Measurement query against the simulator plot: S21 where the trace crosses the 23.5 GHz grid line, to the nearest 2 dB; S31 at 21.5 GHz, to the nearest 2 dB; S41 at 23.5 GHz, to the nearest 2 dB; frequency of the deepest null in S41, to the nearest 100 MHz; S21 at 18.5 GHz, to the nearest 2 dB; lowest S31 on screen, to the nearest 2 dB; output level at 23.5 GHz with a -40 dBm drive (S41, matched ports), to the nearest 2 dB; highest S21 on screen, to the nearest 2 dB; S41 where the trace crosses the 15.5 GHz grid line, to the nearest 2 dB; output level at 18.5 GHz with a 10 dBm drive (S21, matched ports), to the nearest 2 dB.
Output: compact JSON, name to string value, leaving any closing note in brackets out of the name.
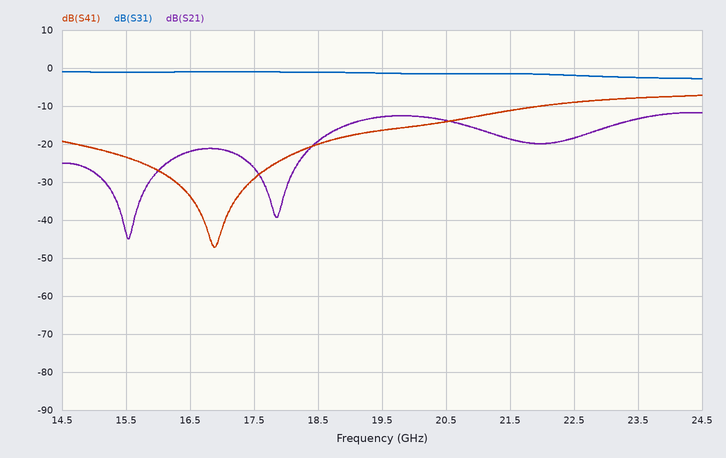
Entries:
{"S21 where the trace crosses the 23.5 GHz grid line, to the nearest 2 dB": "-14 dB", "S31 at 21.5 GHz, to the nearest 2 dB": "-2 dB", "S41 at 23.5 GHz, to the nearest 2 dB": "-8 dB", "frequency of the deepest null in S41, to the nearest 100 MHz": "16.9 GHz", "S21 at 18.5 GHz, to the nearest 2 dB": "-20 dB", "lowest S31 on screen, to the nearest 2 dB": "-2 dB", "output level at 23.5 GHz with a -40 dBm drive (S41, matched ports), to the nearest 2 dB": "-48 dBm", "highest S21 on screen, to the nearest 2 dB": "-12 dB", "S41 where the trace crosses the 15.5 GHz grid line, to the nearest 2 dB": "-24 dB", "output level at 18.5 GHz with a 10 dBm drive (S21, matched ports), to the nearest 2 dB": "-10 dBm"}
